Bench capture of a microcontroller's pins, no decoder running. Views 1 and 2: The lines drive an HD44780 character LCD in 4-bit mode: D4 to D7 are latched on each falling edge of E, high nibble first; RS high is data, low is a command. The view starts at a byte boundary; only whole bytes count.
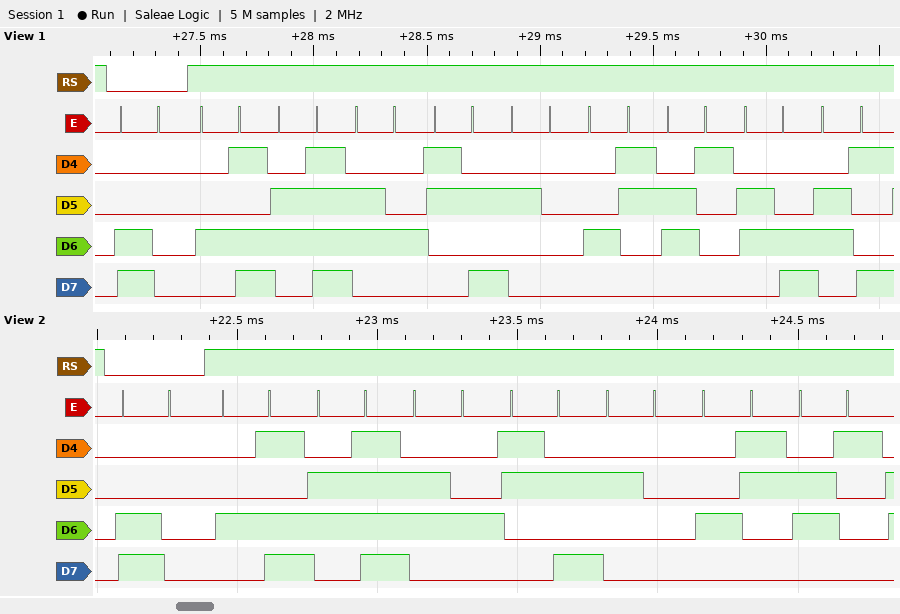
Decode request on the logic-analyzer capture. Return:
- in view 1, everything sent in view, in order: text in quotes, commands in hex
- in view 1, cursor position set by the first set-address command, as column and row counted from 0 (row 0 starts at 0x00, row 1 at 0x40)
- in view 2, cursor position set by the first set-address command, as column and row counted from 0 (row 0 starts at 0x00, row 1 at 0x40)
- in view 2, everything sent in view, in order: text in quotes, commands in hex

0xC0 "Mod: Cali"
column 0, row 1
column 0, row 1
0xC0 "Mod: Ca"
